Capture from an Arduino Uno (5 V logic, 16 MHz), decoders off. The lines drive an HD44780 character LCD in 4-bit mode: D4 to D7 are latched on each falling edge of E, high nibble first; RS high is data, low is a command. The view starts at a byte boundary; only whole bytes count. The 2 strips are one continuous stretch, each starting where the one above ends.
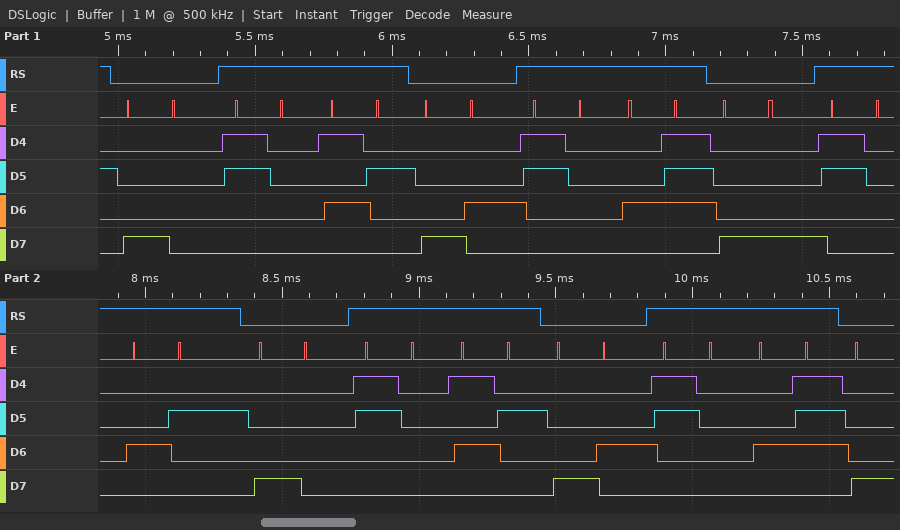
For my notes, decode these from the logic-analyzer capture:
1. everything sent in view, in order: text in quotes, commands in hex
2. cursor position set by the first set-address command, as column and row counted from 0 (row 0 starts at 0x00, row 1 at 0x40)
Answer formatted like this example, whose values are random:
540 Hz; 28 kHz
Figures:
0x80 "0R" 0x84 "0G" 0x88 "0B" 0x80 "0R" 0x84 "0G"; column 0, row 0
